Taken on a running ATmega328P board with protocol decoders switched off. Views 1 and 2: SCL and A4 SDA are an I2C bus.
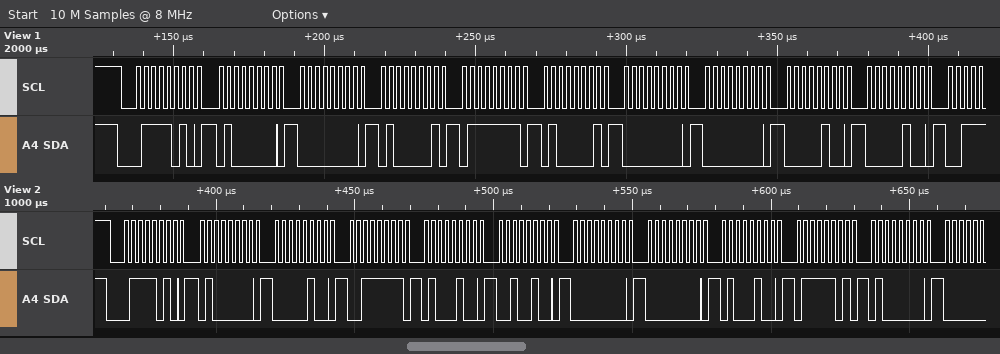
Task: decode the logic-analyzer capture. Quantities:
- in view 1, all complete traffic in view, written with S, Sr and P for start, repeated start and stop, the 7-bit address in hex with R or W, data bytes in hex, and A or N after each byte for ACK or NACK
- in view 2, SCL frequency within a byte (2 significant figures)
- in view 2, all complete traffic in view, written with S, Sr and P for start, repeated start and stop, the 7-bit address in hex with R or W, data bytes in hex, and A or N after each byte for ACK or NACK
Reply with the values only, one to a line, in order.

S 3DW A 40 A 00 A 41 A 7F A 41 A 00 A 00 A 04 A 04 A
400 kHz
S 3DW A 40 A 04 A 3F A 44 A 24 A 00 A 00 A 44 A 7D A 40 A
